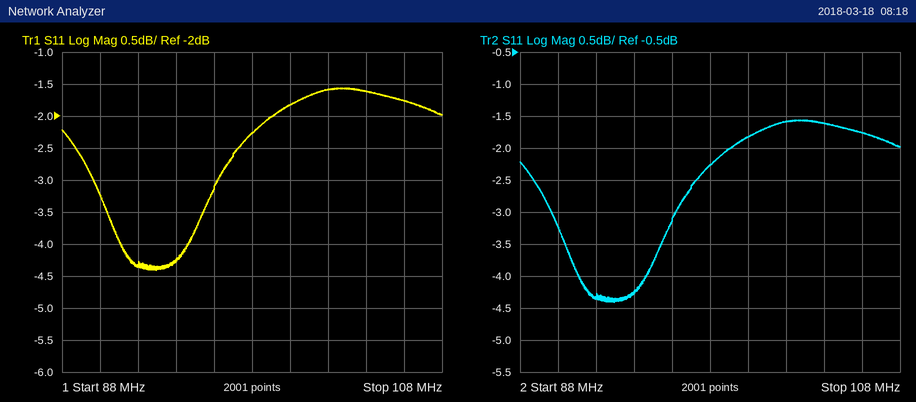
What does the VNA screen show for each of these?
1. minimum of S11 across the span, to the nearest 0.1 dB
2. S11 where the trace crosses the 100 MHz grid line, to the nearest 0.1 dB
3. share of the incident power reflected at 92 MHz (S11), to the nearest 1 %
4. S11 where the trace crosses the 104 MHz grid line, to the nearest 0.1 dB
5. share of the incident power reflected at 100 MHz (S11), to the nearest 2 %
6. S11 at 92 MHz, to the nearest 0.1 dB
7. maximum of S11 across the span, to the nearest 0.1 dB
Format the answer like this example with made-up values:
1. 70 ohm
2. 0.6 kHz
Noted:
1. -4.4 dB
2. -1.8 dB
3. 37 %
4. -1.6 dB
5. 66 %
6. -4.3 dB
7. -1.6 dB
